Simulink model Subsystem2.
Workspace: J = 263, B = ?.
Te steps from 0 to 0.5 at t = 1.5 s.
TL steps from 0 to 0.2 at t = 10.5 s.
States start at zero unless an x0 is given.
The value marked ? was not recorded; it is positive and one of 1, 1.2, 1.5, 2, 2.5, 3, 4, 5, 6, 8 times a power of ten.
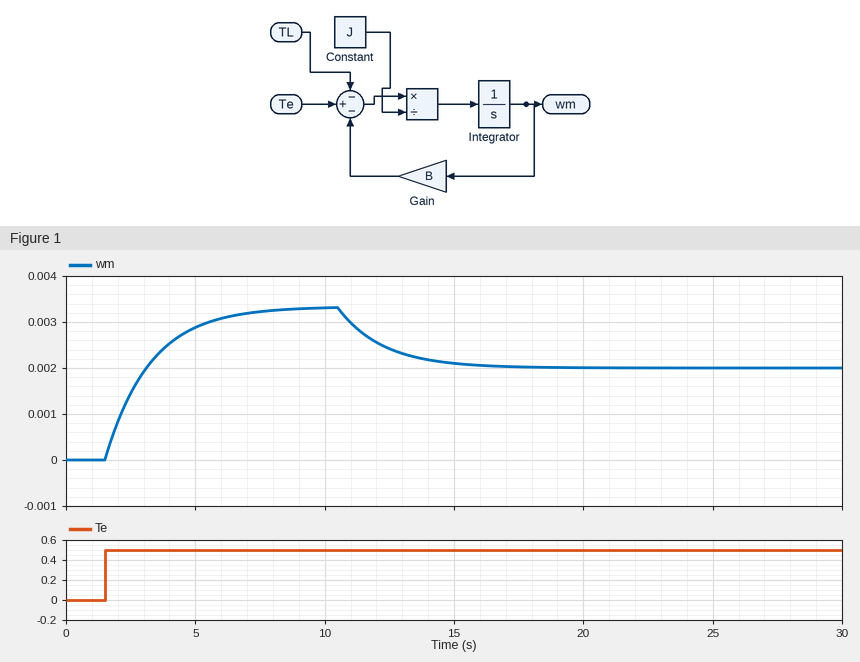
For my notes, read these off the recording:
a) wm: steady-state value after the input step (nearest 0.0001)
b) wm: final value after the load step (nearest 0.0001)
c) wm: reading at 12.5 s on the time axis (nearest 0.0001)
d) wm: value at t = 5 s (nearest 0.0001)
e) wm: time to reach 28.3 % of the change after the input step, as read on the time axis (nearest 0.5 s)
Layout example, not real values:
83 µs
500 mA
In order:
0.0033
0.0020
0.0024
0.0029
2.0 s
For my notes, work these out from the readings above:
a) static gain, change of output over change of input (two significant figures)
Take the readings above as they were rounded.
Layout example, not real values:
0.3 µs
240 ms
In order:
0.0066
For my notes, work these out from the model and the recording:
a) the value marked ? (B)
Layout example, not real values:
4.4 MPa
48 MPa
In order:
150
